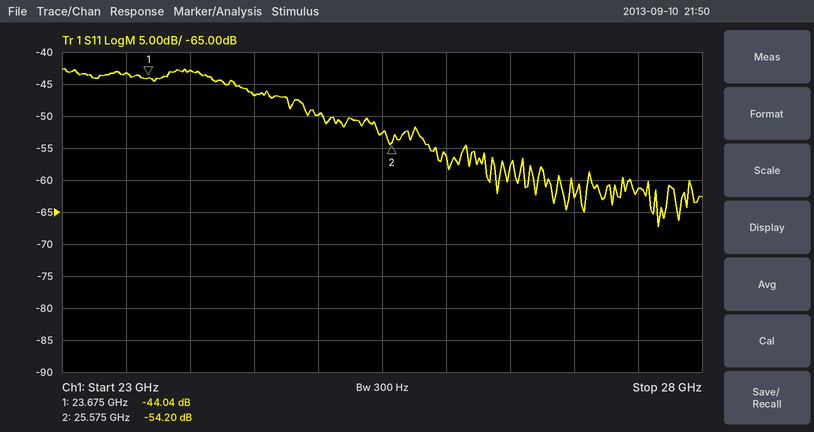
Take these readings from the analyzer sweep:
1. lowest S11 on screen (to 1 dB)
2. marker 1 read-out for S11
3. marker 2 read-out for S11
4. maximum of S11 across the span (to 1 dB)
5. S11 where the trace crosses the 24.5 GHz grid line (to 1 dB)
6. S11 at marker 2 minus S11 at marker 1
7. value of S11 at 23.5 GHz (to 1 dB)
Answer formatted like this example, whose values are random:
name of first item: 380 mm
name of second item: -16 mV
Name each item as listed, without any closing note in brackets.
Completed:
lowest S11 on screen: -67 dB
marker 1 read-out for S11: -44.04 dB
marker 2 read-out for S11: -54.20 dB
maximum of S11 across the span: -43 dB
S11 where the trace crosses the 24.5 GHz grid line: -47 dB
S11 at marker 2 minus S11 at marker 1: -10.16 dB
value of S11 at 23.5 GHz: -43 dB
